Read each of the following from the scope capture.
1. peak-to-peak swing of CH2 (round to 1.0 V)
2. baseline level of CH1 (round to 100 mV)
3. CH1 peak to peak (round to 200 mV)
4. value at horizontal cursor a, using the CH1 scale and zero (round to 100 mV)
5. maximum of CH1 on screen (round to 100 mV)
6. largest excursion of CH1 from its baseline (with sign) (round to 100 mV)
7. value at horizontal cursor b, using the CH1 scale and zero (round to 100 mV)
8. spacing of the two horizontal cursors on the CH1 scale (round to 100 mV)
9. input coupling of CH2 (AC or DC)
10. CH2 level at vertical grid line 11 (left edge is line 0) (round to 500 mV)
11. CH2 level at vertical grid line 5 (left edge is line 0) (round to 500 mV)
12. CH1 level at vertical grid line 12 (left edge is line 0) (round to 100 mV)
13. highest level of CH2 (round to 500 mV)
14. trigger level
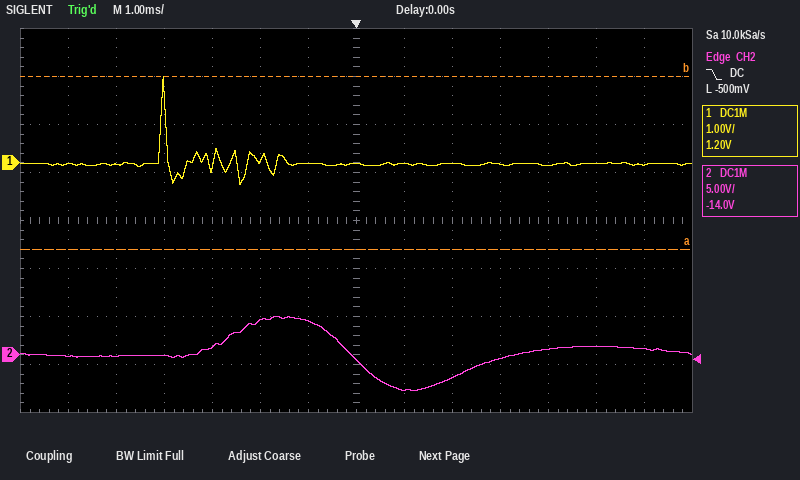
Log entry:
8.0 V
0.0 V
2.2 V
-1.8 V
1.8 V
+1.8 V
1.8 V
3.6 V
DC
500 mV
3.5 V
0.0 V
4.0 V
-500 mV
